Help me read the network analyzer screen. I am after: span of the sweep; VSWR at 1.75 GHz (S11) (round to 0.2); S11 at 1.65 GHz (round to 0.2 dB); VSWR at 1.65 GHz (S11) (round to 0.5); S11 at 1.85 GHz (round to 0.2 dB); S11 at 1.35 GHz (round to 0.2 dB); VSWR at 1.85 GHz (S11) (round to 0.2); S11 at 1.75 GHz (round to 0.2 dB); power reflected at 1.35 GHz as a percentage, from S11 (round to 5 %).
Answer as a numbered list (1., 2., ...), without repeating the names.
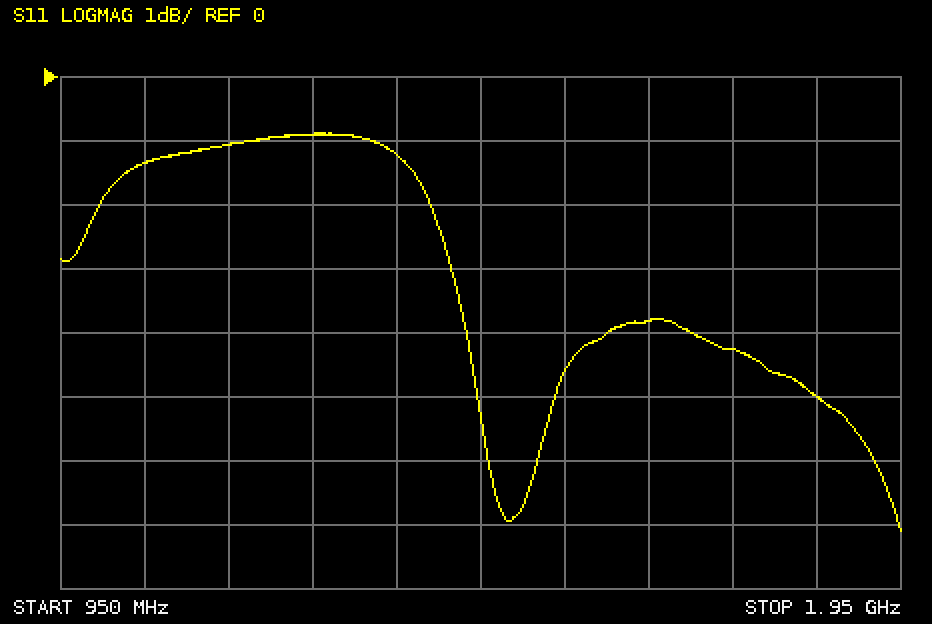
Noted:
1. 1 GHz
2. 4.2
3. -3.8 dB
4. 4.5
5. -5.0 dB
6. -1.2 dB
7. 3.6
8. -4.2 dB
9. 75 %
